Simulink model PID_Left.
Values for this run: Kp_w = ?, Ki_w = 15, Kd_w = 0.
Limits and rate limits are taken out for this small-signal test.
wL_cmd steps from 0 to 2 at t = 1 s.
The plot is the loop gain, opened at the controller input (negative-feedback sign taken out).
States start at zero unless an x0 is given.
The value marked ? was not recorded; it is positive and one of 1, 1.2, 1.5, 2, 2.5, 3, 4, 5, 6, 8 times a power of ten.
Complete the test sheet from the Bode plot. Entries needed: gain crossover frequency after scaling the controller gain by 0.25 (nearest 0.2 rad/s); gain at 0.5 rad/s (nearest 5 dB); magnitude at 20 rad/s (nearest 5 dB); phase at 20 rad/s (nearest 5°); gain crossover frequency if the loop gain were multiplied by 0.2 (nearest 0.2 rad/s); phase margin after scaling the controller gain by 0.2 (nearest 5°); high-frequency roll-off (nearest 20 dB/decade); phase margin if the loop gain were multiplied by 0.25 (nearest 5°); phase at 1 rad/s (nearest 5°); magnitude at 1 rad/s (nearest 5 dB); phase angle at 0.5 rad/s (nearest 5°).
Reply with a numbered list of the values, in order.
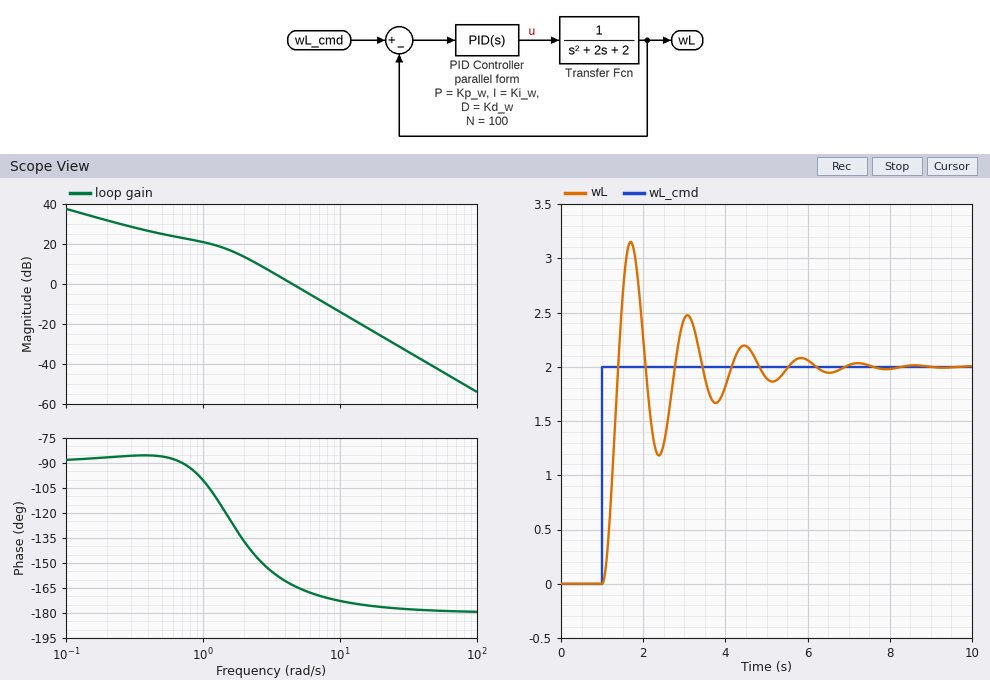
1. 2.2 rad/s
2. 25 dB
3. -25 dB
4. -175°
5. 2.0 rad/s
6. 45°
7. -40 dB/decade
8. 40°
9. -100°
10. 20 dB
11. -85°
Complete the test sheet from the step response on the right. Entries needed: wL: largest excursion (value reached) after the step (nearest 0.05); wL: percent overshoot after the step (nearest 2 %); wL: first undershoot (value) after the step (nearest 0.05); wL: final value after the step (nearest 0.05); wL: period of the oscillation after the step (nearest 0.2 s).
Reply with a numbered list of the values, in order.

1. 3.15
2. 58 %
3. 1.20
4. 2.00
5. 1.4 s
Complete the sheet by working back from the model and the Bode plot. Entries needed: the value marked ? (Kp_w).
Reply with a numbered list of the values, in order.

1. 20
